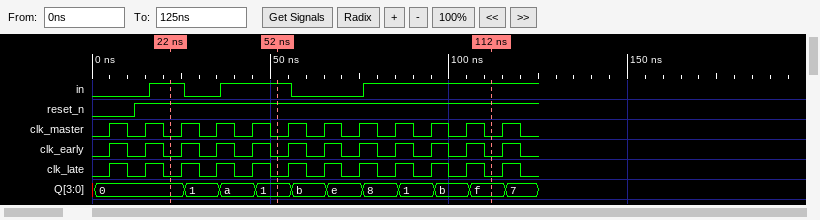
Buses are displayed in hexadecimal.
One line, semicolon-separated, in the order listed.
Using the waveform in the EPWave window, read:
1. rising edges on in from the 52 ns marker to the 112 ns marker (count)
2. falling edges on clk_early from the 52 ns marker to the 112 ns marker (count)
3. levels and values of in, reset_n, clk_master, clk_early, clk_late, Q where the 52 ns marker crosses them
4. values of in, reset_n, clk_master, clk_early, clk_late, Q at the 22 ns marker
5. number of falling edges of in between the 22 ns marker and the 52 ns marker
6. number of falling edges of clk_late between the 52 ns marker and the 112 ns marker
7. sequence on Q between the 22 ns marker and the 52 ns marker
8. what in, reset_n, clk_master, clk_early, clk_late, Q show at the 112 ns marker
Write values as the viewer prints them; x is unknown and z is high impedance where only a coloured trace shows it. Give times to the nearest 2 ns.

1; 6; in=1, reset_n=1, clk_master=0, clk_early=0, clk_late=0, Q=1; in=1, reset_n=1, clk_master=0, clk_early=0, clk_late=0, Q=0; 1; 6; 0, 1, a, 1; in=1, reset_n=1, clk_master=0, clk_early=0, clk_late=0, Q=f
